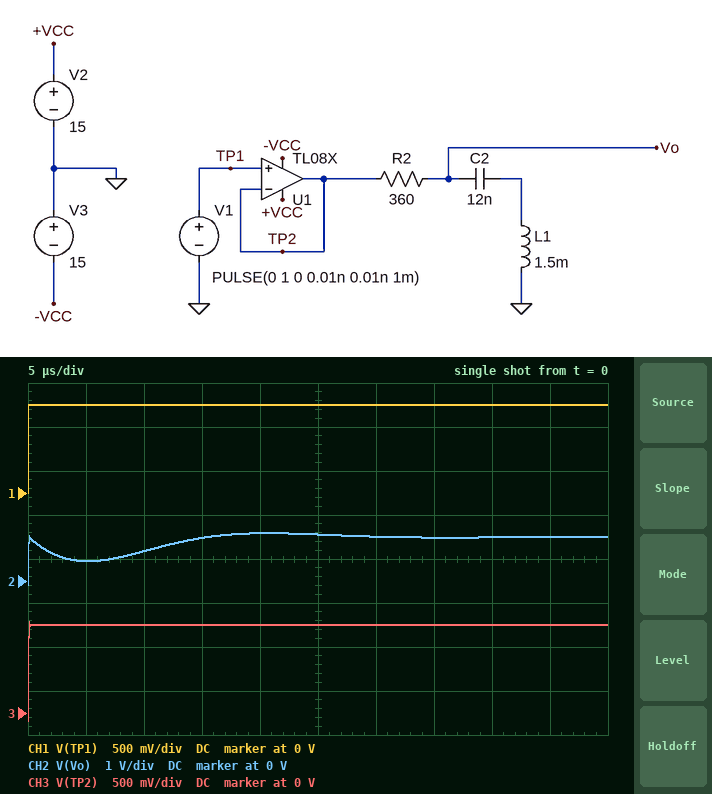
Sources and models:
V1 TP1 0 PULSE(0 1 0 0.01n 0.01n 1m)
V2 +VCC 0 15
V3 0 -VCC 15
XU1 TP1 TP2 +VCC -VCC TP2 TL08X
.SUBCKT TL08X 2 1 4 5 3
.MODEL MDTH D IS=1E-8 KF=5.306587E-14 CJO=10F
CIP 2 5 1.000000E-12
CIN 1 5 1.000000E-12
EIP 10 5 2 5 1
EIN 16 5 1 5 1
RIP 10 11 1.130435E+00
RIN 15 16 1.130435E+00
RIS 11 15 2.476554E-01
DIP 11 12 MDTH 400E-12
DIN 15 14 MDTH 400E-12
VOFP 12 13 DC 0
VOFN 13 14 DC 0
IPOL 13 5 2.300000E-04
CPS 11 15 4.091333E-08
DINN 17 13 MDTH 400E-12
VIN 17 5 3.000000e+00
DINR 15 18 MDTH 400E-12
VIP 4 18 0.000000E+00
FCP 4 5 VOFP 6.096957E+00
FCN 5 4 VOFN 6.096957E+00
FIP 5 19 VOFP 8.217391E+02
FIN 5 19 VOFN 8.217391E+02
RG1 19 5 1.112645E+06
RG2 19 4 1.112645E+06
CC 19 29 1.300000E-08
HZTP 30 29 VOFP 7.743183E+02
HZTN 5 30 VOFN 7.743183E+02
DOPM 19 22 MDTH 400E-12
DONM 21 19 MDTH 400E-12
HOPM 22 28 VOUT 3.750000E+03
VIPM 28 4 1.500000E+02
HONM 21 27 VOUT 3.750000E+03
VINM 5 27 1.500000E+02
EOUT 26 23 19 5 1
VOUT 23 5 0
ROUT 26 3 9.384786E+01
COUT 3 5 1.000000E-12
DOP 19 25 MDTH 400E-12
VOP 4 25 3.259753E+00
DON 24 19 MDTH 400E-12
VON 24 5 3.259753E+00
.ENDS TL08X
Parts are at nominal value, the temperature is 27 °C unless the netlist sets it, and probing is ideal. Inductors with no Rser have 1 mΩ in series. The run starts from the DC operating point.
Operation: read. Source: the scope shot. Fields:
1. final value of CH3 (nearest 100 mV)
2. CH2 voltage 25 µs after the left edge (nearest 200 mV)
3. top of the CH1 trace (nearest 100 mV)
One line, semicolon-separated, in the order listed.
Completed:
1.0 V; 1.0 V; 1.0 V
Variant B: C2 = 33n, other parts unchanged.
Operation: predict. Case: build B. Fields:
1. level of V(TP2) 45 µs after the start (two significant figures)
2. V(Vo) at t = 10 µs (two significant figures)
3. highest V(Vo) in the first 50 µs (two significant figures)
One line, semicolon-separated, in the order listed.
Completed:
1.0 V; 340 mV; 1.0 V
